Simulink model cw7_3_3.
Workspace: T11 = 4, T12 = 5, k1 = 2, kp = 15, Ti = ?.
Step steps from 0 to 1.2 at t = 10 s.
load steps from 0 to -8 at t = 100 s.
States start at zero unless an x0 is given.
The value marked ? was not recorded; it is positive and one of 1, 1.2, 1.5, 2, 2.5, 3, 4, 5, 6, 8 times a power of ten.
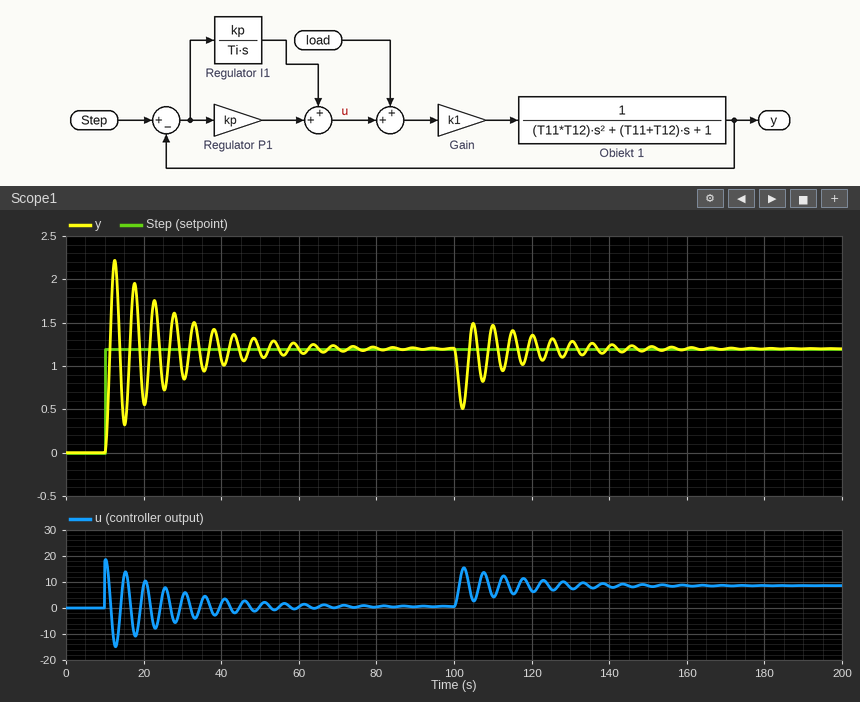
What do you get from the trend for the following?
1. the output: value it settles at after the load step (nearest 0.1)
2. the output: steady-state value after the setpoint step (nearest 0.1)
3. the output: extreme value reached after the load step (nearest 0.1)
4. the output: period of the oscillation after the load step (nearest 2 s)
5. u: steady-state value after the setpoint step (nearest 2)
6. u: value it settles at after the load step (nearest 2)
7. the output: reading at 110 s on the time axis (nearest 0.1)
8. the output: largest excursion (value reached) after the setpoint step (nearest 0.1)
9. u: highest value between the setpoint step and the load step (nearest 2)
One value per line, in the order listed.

1.2
1.2
0.5
6 s
0
8
1.5
2.2
18
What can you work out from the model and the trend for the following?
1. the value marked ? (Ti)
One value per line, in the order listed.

3
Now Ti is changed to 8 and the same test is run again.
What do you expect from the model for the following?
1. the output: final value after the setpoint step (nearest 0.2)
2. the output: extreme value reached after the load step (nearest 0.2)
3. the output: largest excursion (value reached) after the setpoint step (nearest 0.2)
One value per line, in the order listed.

1.2
0.4
2.0
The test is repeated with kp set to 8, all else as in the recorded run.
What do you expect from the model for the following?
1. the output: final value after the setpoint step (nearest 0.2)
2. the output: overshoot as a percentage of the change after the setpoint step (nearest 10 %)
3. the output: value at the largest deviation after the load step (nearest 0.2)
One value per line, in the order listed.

1.2
80 %
0.0
